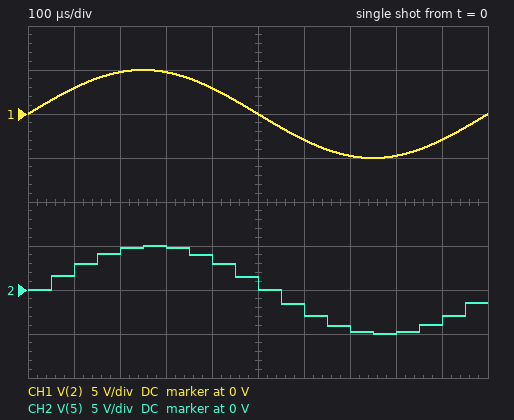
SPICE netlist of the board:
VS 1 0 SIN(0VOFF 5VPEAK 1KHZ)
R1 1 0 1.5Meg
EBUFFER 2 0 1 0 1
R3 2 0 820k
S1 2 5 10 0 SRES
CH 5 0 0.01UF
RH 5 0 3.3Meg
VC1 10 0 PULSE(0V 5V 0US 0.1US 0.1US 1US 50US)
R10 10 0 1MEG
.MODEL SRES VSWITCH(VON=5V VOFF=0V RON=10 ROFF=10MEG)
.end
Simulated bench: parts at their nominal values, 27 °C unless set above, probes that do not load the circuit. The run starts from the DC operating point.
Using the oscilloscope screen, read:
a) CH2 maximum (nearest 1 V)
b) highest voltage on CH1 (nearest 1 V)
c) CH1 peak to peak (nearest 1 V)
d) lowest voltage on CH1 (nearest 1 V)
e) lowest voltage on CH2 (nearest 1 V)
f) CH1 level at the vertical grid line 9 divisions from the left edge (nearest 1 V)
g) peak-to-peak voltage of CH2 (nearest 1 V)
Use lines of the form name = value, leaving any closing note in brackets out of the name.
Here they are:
CH2 maximum = 5 V
highest voltage on CH1 = 5 V
CH1 peak to peak = 10 V
lowest voltage on CH1 = -5 V
lowest voltage on CH2 = -5 V
CH1 level at the vertical grid line 9 divisions from the left edge = -3 V
peak-to-peak voltage of CH2 = 10 V
